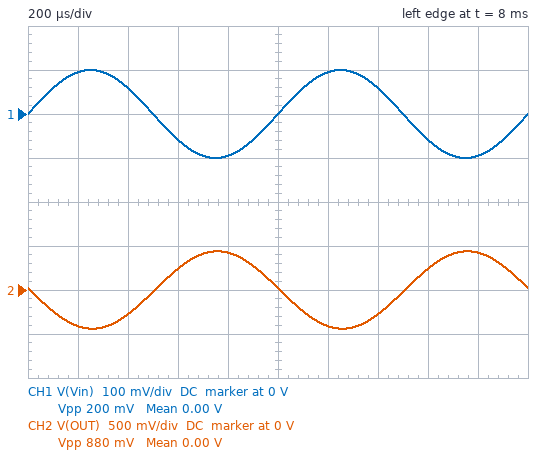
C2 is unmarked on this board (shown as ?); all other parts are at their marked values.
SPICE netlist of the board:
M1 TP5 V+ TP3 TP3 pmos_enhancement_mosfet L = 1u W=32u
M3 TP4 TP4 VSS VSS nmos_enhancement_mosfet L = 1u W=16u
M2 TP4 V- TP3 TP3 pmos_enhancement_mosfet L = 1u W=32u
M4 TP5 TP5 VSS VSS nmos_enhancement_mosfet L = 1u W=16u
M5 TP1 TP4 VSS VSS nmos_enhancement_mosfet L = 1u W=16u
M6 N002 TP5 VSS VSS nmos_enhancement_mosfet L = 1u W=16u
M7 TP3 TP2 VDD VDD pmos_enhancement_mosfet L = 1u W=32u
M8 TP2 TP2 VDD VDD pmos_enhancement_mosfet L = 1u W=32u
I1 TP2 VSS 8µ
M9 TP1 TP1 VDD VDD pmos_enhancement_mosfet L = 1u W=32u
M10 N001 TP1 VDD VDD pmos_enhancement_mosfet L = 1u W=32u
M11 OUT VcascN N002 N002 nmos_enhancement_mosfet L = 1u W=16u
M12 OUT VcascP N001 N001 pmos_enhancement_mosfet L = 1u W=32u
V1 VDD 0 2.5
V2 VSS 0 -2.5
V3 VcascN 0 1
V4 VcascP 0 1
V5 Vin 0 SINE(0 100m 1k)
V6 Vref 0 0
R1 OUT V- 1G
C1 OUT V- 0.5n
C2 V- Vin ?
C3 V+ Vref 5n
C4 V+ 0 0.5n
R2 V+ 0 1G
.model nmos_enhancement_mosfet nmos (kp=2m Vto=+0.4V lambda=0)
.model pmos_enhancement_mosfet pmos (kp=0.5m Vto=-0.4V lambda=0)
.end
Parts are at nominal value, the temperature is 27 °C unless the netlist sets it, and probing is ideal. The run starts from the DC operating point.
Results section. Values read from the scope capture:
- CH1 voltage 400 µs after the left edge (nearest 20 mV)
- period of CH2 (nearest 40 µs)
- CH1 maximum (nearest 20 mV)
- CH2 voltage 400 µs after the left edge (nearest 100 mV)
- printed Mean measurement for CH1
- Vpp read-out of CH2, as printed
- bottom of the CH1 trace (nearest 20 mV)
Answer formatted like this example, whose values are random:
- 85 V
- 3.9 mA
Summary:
- 60 mV
- 1.00 ms
- 100 mV
- -300 mV
- 0.00 V
- 880 mV
- -100 mV
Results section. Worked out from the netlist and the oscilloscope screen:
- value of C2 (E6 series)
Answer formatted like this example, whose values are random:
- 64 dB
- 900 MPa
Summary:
- 2.2 nF
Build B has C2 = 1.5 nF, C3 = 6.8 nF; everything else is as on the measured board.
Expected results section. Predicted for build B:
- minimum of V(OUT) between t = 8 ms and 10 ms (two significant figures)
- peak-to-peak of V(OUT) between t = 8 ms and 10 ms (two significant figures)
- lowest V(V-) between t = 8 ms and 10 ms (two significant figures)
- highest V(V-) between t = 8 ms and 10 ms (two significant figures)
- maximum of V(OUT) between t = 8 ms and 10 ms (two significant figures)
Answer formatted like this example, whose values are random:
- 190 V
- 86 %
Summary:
- -300 mV
- 600 mV
- -2.6 mV
- 2.6 mV
- 300 mV
